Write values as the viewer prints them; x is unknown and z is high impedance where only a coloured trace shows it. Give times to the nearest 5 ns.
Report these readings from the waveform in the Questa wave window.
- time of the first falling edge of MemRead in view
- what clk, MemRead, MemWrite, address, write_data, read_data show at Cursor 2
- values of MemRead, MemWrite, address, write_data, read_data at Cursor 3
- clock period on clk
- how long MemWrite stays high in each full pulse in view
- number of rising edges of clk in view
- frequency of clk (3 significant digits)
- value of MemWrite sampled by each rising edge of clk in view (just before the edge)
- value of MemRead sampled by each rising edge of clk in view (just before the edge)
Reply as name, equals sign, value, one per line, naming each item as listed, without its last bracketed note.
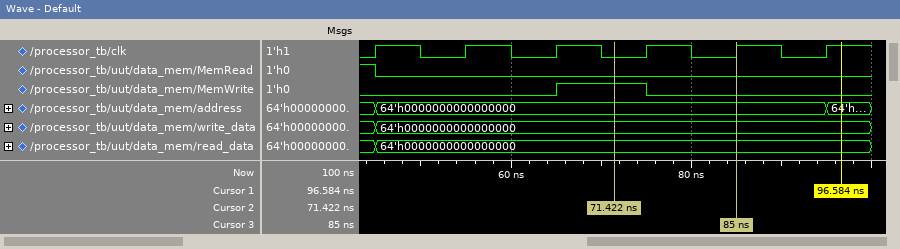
time of the first falling edge of MemRead in view = 45 ns
what clk, MemRead, MemWrite, address, write_data, read_data show at Cursor 2 = clk=0, MemRead=0, MemWrite=1, address=64'h0000000000000000, write_data=64'h0000000000000000, read_data=64'h0000000000000000
values of MemRead, MemWrite, address, write_data, read_data at Cursor 3 = MemRead=0, MemWrite=0, address=64'h0000000000000000, write_data=64'h0000000000000000, read_data=64'h0000000000000000
clock period on clk = 10 ns
how long MemWrite stays high in each full pulse in view = 10 ns
number of rising edges of clk in view = 6
frequency of clk = 100 MHz
value of MemWrite sampled by each rising edge of clk in view = 0 0 0 1 0 0
value of MemRead sampled by each rising edge of clk in view = 1 0 0 0 0 0
